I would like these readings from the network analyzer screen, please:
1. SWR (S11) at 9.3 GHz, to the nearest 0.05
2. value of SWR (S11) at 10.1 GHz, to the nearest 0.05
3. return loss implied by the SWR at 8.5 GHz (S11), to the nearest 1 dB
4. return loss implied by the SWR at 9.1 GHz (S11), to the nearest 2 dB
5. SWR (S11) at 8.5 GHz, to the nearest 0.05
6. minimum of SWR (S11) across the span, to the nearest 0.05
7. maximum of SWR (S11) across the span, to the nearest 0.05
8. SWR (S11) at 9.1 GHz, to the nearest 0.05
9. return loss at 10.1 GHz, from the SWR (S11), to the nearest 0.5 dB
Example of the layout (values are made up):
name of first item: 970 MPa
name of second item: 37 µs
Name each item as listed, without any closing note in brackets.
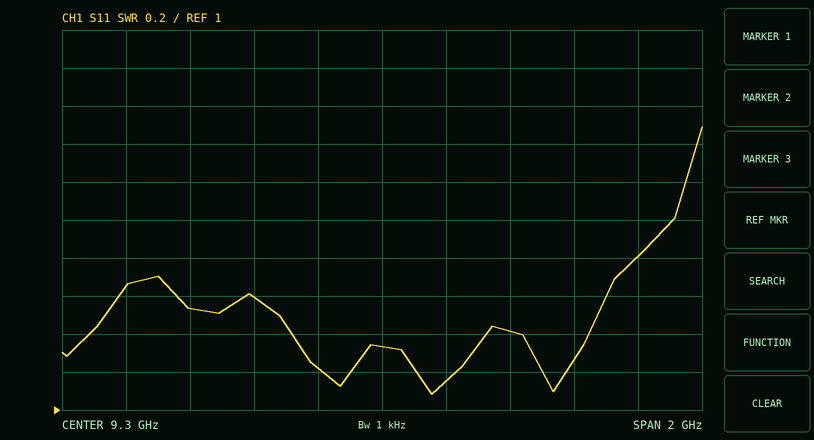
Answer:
SWR (S11) at 9.3 GHz, to the nearest 0.05: 1.35
value of SWR (S11) at 10.1 GHz, to the nearest 0.05: 1.80
return loss implied by the SWR at 8.5 GHz (S11), to the nearest 1 dB: 12 dB
return loss implied by the SWR at 9.1 GHz (S11), to the nearest 2 dB: 20 dB
SWR (S11) at 8.5 GHz, to the nearest 0.05: 1.65
minimum of SWR (S11) across the span, to the nearest 0.05: 1.10
maximum of SWR (S11) across the span, to the nearest 0.05: 2.50
SWR (S11) at 9.1 GHz, to the nearest 0.05: 1.20
return loss at 10.1 GHz, from the SWR (S11), to the nearest 0.5 dB: 11.0 dB
